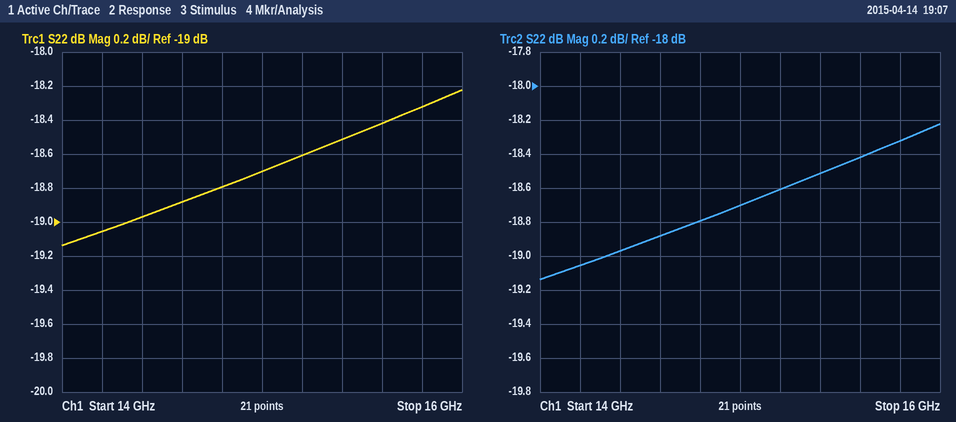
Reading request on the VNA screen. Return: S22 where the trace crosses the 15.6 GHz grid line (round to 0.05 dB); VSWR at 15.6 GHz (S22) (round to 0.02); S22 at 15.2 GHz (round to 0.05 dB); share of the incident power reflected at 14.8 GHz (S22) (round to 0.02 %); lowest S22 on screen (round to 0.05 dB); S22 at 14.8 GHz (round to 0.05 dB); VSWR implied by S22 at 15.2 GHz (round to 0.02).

-18.40 dB
1.28
-18.60 dB
1.32 %
-19.15 dB
-18.80 dB
1.26
